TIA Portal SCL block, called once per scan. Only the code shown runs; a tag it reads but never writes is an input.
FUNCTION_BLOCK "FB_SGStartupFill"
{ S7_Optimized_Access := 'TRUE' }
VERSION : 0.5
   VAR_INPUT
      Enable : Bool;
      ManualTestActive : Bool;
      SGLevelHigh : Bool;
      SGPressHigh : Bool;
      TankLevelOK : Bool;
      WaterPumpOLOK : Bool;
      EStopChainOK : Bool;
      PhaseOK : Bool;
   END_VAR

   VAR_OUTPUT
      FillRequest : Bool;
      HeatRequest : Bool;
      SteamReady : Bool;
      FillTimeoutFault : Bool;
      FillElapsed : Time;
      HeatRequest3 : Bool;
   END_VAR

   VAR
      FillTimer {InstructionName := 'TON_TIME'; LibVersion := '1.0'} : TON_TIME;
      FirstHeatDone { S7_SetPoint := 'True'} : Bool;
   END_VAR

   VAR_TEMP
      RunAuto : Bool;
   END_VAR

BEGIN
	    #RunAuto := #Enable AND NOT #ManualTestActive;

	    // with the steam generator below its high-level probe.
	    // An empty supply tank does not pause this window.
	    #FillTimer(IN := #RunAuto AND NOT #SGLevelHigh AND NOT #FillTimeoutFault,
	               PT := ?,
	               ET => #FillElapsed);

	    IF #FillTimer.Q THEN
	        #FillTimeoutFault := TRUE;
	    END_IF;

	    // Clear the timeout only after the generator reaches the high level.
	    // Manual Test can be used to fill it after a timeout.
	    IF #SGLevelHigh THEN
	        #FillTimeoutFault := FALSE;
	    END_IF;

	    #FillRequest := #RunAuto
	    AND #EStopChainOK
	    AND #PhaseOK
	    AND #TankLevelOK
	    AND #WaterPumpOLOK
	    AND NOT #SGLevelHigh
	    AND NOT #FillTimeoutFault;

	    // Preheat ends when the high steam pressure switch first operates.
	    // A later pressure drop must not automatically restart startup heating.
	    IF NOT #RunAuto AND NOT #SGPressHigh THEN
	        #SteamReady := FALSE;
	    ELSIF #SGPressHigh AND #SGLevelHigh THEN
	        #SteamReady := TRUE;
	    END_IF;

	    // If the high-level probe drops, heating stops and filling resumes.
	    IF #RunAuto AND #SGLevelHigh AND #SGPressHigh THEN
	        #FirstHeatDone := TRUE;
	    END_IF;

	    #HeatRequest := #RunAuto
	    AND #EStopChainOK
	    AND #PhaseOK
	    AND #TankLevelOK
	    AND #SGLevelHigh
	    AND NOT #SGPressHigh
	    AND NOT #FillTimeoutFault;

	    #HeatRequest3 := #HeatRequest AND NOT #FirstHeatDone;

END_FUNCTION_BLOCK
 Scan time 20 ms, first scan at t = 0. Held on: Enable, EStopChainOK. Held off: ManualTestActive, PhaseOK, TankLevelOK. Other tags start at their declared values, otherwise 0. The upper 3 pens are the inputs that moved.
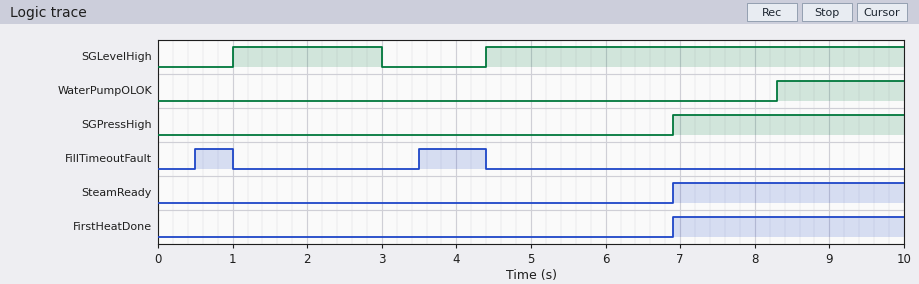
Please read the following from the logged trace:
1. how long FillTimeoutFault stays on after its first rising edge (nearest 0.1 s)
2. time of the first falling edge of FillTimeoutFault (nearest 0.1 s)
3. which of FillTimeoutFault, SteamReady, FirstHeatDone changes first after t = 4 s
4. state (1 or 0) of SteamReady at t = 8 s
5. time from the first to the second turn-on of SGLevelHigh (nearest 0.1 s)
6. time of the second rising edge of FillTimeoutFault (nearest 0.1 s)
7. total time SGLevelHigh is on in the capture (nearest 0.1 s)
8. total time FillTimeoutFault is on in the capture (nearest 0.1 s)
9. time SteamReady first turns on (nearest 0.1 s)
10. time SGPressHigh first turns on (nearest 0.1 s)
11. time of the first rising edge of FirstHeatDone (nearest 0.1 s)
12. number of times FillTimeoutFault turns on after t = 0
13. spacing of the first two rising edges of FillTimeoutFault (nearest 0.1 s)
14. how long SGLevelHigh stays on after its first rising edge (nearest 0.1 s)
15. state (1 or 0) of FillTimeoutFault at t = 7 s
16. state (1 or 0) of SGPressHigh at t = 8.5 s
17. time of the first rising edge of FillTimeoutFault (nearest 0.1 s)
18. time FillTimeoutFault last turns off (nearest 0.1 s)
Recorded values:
0.5 s
1.0 s
FillTimeoutFault
1
3.4 s
3.5 s
7.6 s
1.4 s
6.9 s
6.9 s
6.9 s
2
3.0 s
2.0 s
0
1
0.5 s
4.4 s
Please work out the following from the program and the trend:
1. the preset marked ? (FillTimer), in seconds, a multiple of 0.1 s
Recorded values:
0.5 s
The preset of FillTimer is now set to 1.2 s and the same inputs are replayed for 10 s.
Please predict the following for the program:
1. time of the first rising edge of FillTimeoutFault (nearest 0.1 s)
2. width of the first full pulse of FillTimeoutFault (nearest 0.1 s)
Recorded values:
4.2 s
0.2 s
